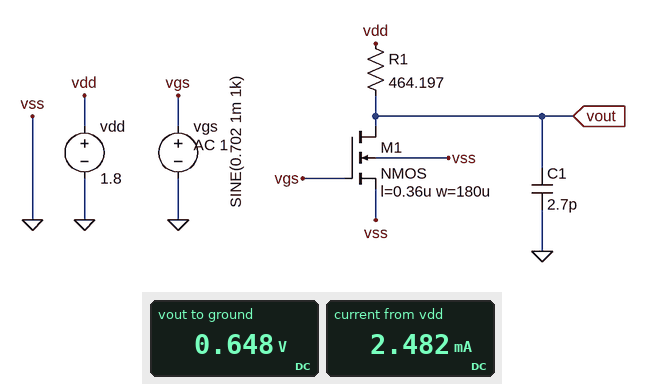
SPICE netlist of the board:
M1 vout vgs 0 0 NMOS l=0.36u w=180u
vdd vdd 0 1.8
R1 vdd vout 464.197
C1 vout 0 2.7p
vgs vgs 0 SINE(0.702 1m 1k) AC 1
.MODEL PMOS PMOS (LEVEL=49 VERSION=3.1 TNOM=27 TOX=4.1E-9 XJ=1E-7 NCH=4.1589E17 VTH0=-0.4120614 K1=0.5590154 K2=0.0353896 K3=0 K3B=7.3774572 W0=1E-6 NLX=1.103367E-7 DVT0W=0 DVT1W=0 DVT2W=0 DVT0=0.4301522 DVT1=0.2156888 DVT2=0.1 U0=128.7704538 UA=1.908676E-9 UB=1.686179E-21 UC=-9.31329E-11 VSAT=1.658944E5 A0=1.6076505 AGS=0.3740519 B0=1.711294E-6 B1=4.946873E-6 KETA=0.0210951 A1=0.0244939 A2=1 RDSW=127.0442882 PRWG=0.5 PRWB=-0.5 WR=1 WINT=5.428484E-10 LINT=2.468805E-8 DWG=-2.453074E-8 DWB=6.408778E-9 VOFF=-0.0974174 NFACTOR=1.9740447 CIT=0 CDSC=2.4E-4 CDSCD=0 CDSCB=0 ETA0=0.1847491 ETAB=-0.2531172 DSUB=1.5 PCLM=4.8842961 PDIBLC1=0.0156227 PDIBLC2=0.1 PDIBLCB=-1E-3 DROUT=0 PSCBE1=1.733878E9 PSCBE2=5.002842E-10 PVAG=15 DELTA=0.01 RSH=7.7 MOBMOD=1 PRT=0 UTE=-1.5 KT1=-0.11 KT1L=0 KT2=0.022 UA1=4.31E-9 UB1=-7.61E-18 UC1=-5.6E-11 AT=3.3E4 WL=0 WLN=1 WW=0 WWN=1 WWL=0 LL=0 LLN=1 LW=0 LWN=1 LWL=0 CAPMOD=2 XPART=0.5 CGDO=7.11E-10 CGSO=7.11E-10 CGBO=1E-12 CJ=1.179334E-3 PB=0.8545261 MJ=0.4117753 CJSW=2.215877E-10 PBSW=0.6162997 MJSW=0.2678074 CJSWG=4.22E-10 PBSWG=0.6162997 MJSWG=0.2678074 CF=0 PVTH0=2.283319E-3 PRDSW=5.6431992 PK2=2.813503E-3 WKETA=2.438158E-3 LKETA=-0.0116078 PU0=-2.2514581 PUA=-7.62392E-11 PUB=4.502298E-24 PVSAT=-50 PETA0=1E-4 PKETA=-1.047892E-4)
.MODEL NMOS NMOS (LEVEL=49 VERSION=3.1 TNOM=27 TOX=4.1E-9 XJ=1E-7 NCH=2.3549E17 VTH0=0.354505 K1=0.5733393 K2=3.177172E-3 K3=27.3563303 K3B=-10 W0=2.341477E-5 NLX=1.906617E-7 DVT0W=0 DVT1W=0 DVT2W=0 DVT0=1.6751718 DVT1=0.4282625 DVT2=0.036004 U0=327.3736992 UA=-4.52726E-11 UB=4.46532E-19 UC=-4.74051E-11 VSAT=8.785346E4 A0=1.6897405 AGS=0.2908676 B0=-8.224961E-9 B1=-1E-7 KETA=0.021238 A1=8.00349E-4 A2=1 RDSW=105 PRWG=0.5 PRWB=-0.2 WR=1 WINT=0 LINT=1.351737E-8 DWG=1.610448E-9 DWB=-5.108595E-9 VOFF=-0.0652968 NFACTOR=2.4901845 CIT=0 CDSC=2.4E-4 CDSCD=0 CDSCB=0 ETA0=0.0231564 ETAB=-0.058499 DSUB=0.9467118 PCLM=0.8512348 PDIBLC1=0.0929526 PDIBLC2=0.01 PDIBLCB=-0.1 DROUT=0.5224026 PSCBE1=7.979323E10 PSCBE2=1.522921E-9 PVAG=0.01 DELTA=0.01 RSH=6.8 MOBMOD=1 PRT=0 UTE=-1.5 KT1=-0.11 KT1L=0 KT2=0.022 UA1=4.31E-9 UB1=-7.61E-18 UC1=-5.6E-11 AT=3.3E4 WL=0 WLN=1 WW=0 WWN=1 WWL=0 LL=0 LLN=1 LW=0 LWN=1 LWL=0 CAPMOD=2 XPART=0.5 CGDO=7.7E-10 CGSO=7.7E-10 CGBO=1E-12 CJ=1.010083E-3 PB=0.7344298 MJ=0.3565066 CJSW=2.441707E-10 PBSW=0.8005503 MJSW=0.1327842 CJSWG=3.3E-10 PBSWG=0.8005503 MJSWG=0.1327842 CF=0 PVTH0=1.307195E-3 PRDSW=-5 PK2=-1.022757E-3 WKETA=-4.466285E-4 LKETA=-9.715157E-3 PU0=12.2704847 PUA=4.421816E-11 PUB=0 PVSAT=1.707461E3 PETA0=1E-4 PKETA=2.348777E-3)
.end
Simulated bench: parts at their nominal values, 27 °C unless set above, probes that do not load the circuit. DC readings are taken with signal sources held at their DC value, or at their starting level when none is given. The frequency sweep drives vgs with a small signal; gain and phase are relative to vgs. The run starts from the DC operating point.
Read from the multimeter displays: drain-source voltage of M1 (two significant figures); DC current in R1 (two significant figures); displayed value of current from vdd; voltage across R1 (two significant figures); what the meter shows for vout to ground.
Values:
650 mV
2.5 mA
2.482 mA
1.2 V
0.648 V
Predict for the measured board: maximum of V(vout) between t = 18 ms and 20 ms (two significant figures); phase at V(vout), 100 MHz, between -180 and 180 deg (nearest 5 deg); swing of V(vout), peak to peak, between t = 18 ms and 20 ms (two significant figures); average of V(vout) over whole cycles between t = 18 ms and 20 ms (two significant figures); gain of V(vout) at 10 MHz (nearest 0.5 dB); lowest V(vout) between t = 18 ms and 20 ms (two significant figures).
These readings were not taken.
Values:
660 mV
140 deg
17 mV
650 mV
18.5 dB
640 mV
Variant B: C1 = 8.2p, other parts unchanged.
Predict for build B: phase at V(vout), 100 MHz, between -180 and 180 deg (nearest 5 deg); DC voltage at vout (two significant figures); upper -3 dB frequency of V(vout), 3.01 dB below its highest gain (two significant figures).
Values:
115 deg
650 mV
45 MHz
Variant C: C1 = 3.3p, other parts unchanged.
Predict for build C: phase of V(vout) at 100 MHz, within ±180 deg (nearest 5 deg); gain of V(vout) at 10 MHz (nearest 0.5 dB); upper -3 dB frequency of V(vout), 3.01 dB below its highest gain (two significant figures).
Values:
135 deg
18.5 dB
110 MHz
